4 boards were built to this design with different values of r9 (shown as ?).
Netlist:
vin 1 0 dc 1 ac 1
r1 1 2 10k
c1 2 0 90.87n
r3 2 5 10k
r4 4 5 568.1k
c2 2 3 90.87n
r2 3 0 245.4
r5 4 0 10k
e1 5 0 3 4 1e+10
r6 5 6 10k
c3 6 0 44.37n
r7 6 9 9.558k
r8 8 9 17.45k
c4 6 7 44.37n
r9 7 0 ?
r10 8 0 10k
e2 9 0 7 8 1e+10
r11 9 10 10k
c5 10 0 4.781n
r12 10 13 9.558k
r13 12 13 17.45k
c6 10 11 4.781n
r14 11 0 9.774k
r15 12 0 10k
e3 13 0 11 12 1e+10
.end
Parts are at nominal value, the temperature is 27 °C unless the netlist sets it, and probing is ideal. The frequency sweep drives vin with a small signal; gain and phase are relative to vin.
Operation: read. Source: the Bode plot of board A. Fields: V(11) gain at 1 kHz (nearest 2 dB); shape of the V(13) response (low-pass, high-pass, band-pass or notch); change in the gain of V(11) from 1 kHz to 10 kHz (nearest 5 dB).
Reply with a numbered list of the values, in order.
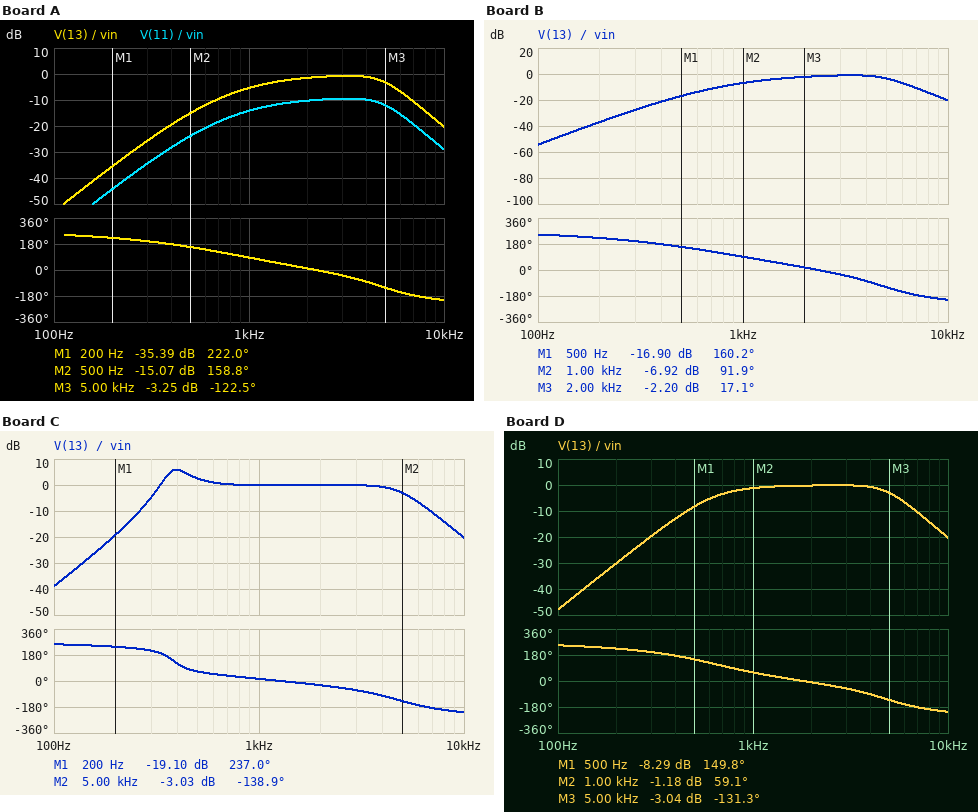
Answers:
1. -14 dB
2. band-pass
3. -15 dB
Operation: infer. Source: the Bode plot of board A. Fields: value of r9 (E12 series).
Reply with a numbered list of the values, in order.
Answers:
1. 3.9 kΩ
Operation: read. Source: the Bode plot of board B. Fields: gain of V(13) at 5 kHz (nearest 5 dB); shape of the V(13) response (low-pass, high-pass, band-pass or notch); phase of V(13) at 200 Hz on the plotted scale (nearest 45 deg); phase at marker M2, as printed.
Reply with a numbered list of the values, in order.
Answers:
1. -5 dB
2. band-pass
3. 225 deg
4. 91.9 deg
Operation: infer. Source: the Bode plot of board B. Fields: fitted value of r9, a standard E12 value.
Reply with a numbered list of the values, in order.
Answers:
1. 3.3 kΩ
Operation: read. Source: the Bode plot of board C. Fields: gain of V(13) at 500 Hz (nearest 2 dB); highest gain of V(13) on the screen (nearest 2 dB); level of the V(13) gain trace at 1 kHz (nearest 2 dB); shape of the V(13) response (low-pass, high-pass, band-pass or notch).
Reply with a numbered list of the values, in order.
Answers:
1. 2 dB
2. 6 dB
3. 0 dB
4. band-pass
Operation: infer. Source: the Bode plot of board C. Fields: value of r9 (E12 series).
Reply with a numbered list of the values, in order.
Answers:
1. 18 kΩ
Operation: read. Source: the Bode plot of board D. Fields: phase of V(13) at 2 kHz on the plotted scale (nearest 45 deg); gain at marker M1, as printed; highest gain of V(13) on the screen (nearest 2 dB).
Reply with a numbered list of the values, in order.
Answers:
1. 0 deg
2. -8.29 dB
3. 0 dB
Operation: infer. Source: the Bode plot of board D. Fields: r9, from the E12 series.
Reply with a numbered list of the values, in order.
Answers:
1. 6.8 kΩ
